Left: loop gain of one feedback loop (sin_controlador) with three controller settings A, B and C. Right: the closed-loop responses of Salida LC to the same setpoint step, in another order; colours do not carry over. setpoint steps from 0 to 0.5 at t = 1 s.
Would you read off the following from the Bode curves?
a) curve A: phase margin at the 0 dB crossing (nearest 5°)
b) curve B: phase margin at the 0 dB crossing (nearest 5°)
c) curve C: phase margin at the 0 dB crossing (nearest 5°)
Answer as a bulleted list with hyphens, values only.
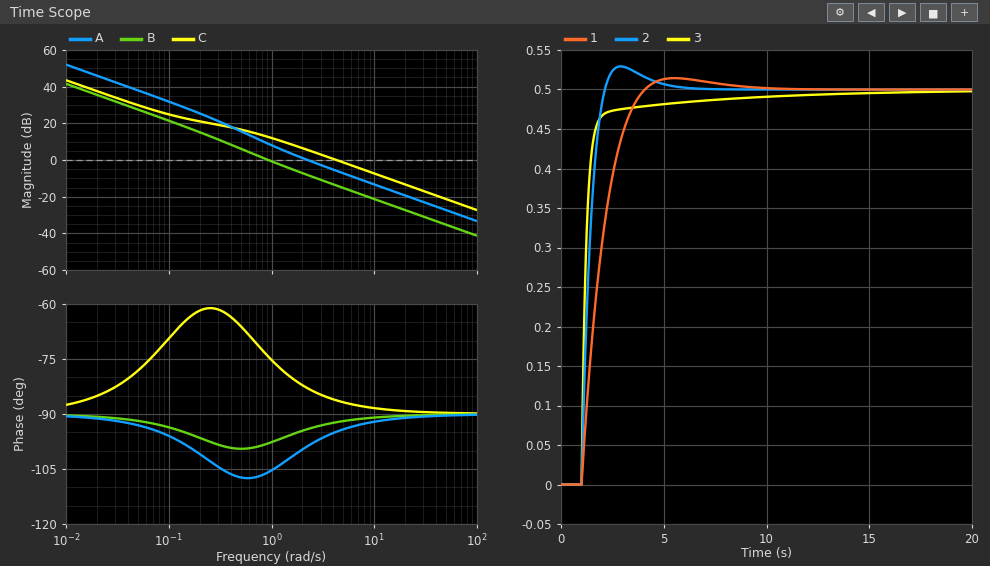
- 80°
- 80°
- 95°
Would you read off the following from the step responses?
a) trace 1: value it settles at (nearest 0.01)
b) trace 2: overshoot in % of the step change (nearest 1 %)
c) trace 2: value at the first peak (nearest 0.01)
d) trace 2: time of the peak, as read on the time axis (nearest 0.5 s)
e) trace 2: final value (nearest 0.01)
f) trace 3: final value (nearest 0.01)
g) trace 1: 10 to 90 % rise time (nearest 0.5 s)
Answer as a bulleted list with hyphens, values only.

- 0.50
- 6 %
- 0.53
- 3.0 s
- 0.50
- 0.50
- 2.0 s
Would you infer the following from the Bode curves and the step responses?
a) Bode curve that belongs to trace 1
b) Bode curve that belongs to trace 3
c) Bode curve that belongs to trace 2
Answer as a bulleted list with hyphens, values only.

- B
- C
- A
